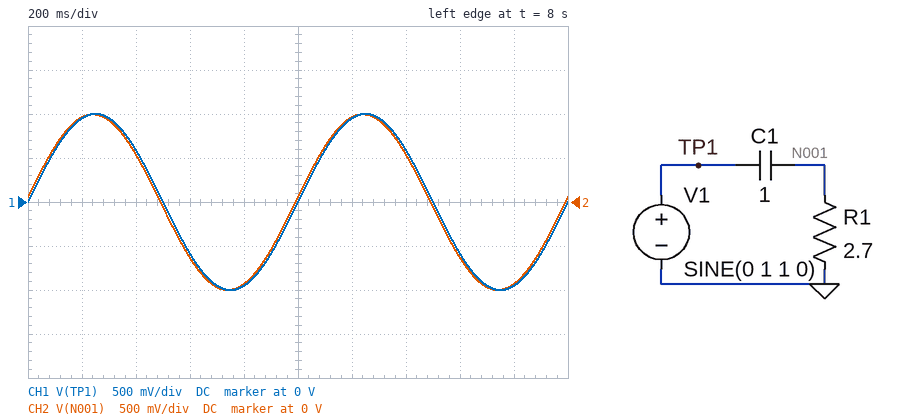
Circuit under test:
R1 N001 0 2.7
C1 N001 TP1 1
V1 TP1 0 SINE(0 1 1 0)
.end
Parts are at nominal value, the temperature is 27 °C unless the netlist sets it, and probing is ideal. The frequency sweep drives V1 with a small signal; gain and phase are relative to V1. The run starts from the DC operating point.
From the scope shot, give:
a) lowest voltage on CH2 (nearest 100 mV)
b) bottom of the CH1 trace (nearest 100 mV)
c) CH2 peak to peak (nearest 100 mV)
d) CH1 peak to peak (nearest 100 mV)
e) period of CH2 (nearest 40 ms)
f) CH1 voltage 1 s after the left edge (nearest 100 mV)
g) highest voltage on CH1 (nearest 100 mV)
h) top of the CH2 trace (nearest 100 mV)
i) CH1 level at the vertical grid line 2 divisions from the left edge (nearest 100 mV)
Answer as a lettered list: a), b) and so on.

a) -1.0 V
b) -1.0 V
c) 2.0 V
d) 2.0 V
e) 1.00 s
f) 0 V
g) 1.0 V
h) 1.0 V
i) 600 mV
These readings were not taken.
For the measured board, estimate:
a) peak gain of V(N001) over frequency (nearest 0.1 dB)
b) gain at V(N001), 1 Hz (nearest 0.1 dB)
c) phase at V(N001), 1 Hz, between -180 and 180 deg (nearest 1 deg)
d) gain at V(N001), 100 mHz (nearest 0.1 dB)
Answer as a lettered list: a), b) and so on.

a) 0 dB
b) 0 dB
c) 3 deg
d) -1.3 dB
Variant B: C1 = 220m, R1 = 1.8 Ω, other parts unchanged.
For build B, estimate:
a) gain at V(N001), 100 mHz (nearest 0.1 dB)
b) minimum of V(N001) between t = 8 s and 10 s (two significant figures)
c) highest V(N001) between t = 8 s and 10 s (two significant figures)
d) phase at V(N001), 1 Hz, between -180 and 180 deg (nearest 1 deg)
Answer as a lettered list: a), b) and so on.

a) -12.3 dB
b) -930 mV
c) 930 mV
d) 22 deg
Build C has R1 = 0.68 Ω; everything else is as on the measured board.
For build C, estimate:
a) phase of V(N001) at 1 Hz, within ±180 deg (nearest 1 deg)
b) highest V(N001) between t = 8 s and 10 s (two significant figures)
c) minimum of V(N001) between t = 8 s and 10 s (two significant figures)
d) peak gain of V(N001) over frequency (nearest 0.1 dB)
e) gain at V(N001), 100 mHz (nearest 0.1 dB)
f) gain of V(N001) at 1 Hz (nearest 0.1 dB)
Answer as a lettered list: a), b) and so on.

a) 13 deg
b) 970 mV
c) -970 mV
d) 0 dB
e) -8.1 dB
f) -0.2 dB
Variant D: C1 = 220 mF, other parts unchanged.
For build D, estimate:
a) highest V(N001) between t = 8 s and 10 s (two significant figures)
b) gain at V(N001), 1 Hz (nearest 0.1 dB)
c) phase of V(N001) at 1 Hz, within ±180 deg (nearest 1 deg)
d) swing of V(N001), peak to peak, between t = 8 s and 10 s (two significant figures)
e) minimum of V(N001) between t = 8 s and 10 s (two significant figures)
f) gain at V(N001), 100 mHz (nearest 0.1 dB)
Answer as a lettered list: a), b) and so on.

a) 970 mV
b) -0.3 dB
c) 15 deg
d) 1.9 V
e) -970 mV
f) -9.1 dB
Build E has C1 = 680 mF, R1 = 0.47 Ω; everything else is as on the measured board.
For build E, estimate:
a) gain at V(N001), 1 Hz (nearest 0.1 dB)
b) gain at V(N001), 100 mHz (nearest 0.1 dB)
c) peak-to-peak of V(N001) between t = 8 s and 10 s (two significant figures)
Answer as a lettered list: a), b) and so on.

a) -1.0 dB
b) -14.1 dB
c) 1.8 V
